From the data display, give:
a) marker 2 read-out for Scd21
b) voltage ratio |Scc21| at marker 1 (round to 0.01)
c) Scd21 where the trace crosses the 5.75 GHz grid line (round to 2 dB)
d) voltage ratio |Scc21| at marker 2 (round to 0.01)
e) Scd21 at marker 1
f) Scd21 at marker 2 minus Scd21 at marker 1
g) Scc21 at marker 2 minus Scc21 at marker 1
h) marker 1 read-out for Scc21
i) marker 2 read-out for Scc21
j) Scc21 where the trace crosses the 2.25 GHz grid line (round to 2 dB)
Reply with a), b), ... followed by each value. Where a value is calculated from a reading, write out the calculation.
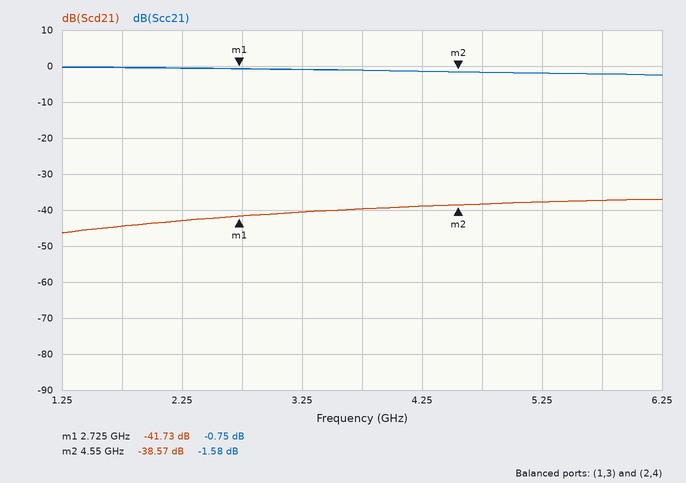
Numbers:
a) -38.57 dB
b) 10^(-0.75/20) ≈ 0.92
c) -38 dB
d) 10^(-1.58/20) ≈ 0.83
e) -41.73 dB
f) -38.57 − (-41.73) = 3.16 dB
g) -1.58 − (-0.75) = -0.83 dB
h) -0.75 dB
i) -1.58 dB
j) 0 dB
